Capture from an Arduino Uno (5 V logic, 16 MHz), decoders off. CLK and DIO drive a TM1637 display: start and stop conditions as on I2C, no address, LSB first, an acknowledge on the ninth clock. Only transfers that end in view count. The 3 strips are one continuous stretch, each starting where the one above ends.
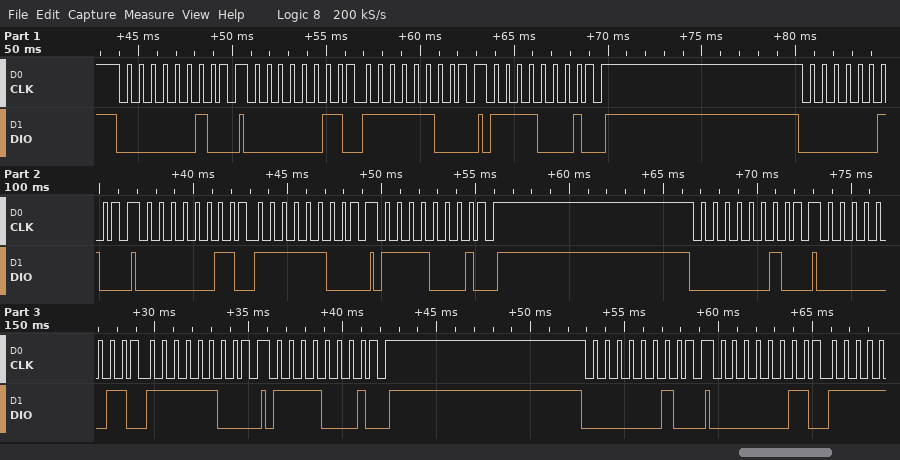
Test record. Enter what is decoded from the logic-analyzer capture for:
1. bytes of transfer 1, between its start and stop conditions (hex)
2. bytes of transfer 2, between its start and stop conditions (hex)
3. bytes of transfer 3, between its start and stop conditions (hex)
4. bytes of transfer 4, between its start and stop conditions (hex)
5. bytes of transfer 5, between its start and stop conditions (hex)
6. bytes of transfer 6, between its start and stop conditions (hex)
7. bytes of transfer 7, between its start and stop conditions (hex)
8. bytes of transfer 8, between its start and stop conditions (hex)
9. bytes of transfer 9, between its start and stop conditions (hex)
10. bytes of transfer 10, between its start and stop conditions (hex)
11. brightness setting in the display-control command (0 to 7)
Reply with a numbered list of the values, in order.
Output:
1. 40
2. C0 3F
3. 8F
4. 40
5. C0 3F
6. 8F
7. 40
8. C0 3F
9. 8F
10. 40
11. 7
